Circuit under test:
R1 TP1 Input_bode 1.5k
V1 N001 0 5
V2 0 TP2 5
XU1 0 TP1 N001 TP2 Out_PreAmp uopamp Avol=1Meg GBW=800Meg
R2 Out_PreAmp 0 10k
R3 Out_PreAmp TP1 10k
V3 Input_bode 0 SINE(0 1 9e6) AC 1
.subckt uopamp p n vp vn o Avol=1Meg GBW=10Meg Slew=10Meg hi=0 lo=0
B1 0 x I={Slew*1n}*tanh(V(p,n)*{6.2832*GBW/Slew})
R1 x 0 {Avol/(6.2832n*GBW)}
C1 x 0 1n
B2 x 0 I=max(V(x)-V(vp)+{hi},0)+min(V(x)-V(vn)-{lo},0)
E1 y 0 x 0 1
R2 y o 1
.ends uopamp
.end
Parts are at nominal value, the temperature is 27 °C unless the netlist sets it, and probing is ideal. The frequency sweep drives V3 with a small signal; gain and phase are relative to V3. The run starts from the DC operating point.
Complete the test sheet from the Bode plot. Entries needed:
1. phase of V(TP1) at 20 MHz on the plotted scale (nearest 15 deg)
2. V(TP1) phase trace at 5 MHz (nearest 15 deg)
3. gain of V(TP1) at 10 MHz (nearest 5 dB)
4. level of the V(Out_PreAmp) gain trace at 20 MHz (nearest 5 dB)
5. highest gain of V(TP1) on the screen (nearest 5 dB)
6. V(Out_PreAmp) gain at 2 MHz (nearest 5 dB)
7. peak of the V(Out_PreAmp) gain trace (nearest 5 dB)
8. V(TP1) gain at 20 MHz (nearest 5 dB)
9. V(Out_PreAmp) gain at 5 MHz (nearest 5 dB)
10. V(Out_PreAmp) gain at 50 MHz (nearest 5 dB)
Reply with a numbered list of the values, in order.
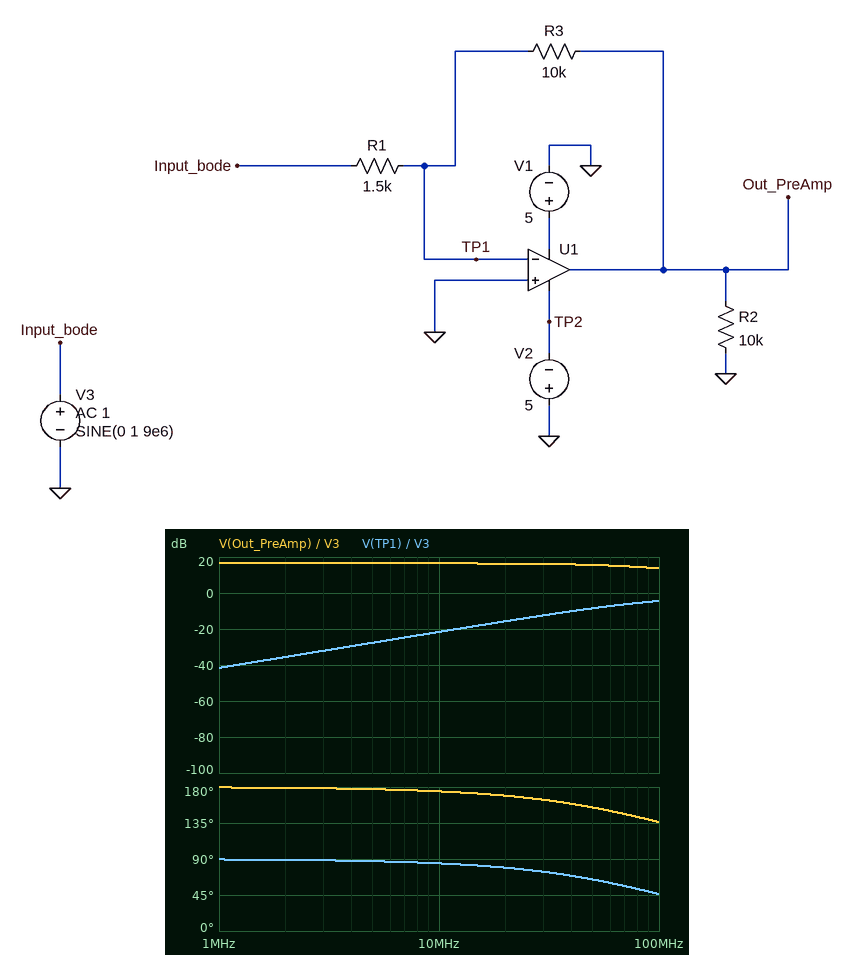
1. 75 deg
2. 90 deg
3. -20 dB
4. 15 dB
5. -5 dB
6. 15 dB
7. 15 dB
8. -15 dB
9. 15 dB
10. 15 dB
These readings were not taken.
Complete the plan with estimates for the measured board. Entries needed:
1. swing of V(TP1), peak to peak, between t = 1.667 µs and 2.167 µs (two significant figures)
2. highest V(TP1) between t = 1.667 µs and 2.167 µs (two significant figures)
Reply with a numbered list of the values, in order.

1. 1.7 V
2. 860 mV
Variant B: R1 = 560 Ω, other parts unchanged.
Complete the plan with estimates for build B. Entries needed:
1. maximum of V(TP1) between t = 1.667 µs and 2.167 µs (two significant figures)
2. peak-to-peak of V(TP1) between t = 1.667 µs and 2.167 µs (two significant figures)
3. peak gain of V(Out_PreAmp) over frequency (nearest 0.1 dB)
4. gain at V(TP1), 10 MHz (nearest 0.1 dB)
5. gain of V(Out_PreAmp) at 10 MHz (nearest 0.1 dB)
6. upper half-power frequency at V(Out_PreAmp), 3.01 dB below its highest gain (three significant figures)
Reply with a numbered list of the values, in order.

1. 940 mV
2. 1.9 V
3. 25.0 dB
4. -13.3 dB
5. 24.8 dB
6. 42.4 MHz
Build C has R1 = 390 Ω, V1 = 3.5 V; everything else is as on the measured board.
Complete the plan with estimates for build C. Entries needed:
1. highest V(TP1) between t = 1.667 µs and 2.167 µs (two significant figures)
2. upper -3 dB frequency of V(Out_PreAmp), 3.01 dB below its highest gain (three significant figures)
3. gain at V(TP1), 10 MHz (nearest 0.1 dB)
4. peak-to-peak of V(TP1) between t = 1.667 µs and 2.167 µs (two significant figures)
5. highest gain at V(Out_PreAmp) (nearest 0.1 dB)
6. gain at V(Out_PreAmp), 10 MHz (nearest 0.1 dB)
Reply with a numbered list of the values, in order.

1. 960 mV
2. 30.0 MHz
3. -10.3 dB
4. 1.9 V
5. 28.2 dB
6. 27.7 dB
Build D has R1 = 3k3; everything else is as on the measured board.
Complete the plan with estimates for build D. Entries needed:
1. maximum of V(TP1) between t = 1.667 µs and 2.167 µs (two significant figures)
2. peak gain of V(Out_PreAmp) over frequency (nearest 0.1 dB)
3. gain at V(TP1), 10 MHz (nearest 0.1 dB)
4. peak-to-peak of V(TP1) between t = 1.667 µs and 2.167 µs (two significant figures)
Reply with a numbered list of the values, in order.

1. 750 mV
2. 9.6 dB
3. -28.4 dB
4. 1.5 V
